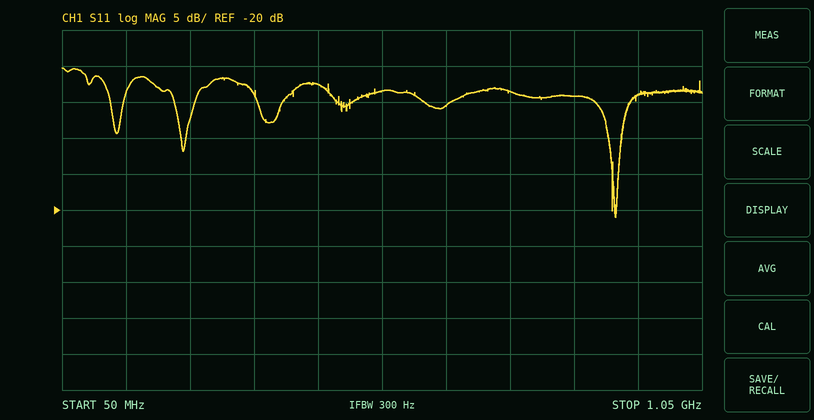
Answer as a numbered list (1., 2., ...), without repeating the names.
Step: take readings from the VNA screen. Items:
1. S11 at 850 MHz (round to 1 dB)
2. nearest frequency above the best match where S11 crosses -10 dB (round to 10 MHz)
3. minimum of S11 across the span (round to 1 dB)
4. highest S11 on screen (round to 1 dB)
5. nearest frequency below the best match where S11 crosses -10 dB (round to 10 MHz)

1. -4 dB
2. 920 MHz
3. -21 dB
4. 0 dB
5. 900 MHz
